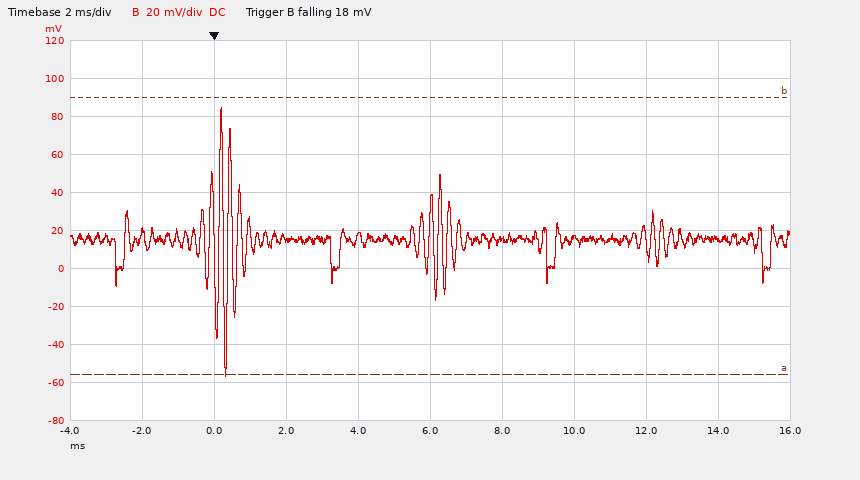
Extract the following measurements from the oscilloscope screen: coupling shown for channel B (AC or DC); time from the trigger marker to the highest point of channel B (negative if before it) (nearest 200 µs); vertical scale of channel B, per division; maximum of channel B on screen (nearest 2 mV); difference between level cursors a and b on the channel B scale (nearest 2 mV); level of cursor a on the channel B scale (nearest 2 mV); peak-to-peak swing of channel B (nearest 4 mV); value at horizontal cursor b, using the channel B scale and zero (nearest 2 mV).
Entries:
DC
+200 µs
20 mV
84 mV
146 mV
-56 mV
140 mV
90 mV
